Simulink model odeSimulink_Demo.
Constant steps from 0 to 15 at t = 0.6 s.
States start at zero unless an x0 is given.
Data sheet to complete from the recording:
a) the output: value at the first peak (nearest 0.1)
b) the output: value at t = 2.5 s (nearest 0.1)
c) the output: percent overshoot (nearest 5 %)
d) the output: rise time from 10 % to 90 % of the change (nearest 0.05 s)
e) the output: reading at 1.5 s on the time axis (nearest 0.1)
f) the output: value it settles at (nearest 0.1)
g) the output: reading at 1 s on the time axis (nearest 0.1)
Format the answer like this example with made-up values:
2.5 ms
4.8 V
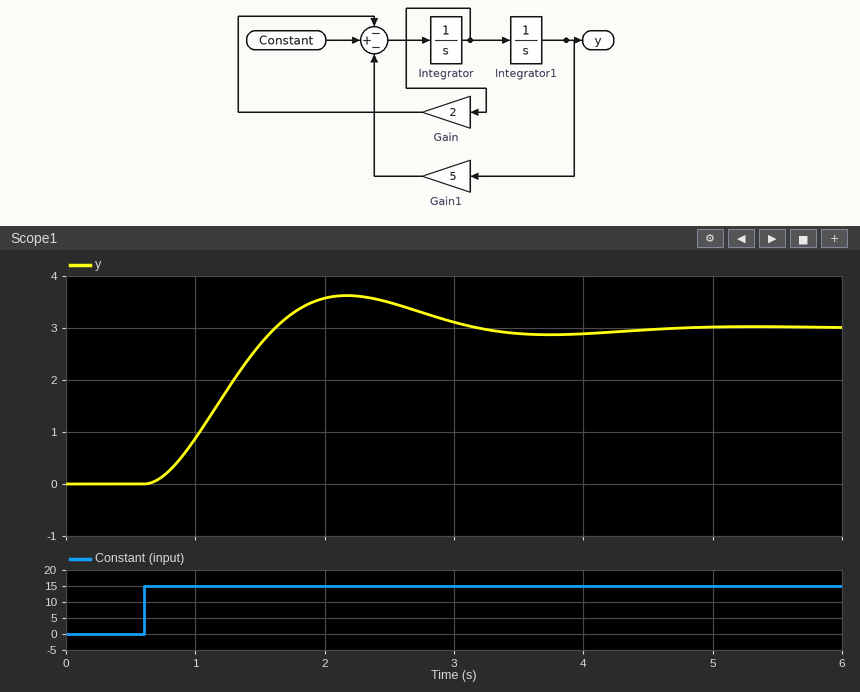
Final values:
3.6
3.5
20 %
0.70 s
2.7
3.0
0.9
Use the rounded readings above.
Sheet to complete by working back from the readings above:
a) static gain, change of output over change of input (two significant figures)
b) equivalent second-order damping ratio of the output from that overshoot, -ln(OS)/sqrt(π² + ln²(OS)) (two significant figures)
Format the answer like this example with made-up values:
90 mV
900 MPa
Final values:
0.20
0.46
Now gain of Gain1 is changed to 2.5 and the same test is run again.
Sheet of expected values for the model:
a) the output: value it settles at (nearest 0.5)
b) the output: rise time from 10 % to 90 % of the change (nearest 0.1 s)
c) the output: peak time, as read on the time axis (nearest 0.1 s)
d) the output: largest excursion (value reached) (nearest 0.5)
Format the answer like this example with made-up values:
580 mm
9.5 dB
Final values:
6.0
1.2 s
3.2 s
6.5
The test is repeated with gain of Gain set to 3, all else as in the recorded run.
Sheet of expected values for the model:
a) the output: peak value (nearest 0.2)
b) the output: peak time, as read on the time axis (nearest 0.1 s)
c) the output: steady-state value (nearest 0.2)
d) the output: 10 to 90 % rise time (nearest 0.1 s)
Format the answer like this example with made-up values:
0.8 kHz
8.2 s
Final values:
3.2
2.5 s
3.0
0.9 s
